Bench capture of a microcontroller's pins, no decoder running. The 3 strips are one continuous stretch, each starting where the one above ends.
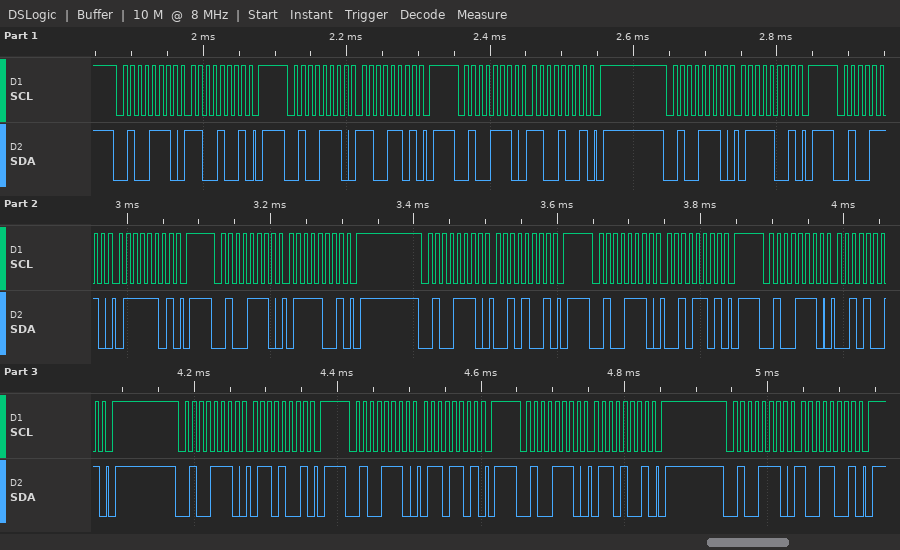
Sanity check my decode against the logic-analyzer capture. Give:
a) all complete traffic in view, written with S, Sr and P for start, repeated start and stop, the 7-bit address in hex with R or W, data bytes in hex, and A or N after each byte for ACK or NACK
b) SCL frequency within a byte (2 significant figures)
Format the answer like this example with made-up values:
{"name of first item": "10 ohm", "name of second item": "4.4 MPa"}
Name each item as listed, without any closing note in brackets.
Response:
{"all complete traffic in view, written with S, Sr and P for start, repeated start and stop, the 7-bit address in hex with R or W, data bytes in hex, and A or N after each byte for ACK or NACK": "S 27W A C9 A P S 27W A CD A P S 27W A C9 A P S 27W A 79 A P S 27W A 7D A P S 27W A 79 A P S 27W A 29 A P S 27W A 2D A P S 27W A 29 A P S 27W A 69 A P S 27W A 6D A P S 27W A 69 A P S 27W A 99 A P", "SCL frequency within a byte": "100 kHz"}
